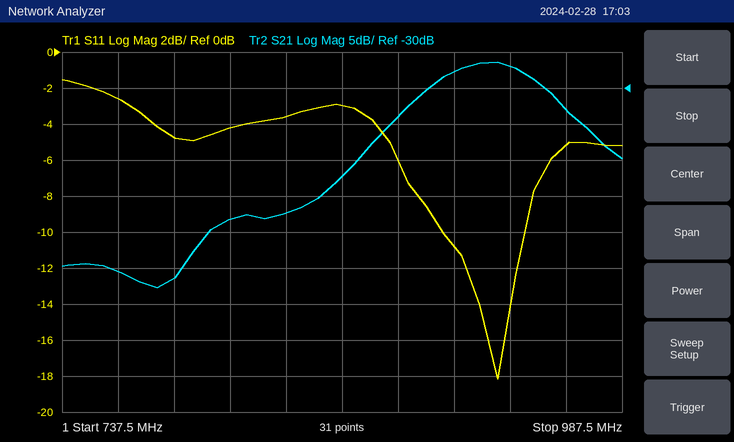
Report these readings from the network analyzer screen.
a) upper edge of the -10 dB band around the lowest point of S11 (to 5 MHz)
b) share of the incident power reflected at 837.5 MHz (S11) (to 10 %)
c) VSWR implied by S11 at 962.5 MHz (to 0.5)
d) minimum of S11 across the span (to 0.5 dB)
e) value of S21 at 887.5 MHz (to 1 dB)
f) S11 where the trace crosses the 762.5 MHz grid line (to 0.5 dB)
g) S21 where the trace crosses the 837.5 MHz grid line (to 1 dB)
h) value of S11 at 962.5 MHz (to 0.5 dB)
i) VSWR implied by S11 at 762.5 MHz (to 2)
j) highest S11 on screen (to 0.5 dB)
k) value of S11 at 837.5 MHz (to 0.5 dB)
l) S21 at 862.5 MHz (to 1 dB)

945 MHz
40 %
3.5
-18.0 dB
-34 dB
-2.5 dB
-47 dB
-5.0 dB
6
-1.5 dB
-3.5 dB
-42 dB
